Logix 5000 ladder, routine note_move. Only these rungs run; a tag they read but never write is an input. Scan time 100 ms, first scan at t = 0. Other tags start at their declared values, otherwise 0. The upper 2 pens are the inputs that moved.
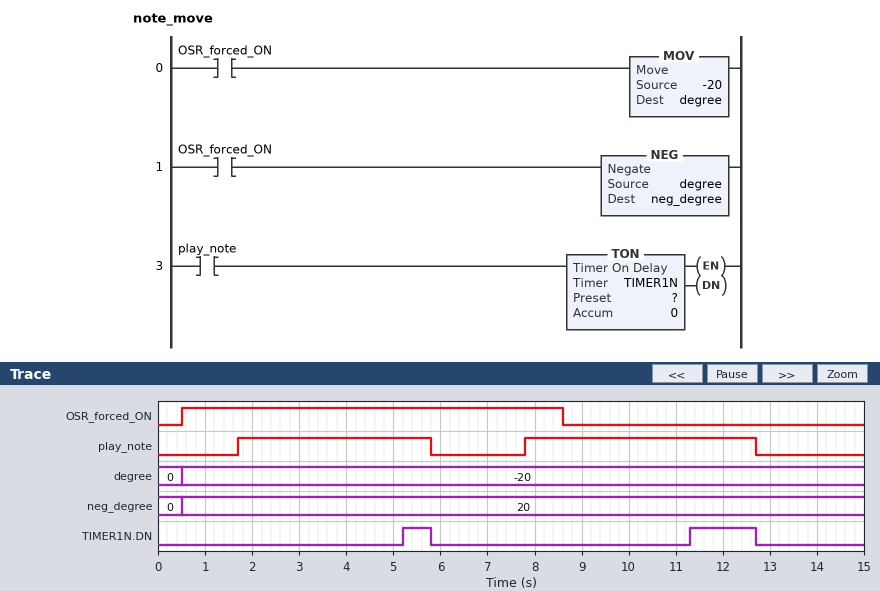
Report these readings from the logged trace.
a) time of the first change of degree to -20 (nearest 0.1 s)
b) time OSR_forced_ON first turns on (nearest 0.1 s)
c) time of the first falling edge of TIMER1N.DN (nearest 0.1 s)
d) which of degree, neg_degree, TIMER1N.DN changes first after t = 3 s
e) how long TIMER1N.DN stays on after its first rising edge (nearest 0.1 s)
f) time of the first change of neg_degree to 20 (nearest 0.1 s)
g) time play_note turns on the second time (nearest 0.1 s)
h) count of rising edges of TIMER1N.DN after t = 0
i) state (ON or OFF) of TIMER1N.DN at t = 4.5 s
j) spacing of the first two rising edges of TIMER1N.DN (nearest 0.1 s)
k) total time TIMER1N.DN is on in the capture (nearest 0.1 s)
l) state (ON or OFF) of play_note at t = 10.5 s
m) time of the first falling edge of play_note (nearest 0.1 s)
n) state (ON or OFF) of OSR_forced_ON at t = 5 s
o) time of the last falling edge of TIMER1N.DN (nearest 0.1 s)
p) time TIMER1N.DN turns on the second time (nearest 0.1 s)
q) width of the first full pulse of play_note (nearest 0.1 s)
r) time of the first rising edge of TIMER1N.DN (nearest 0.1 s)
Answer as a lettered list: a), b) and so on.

a) 0.5 s
b) 0.5 s
c) 5.8 s
d) TIMER1N.DN
e) 0.6 s
f) 0.5 s
g) 7.8 s
h) 2
i) OFF
j) 6.1 s
k) 2.0 s
l) ON
m) 5.8 s
n) ON
o) 12.7 s
p) 11.3 s
q) 4.1 s
r) 5.2 s
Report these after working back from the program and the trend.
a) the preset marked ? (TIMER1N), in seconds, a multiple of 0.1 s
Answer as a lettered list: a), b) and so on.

a) 3.5 s
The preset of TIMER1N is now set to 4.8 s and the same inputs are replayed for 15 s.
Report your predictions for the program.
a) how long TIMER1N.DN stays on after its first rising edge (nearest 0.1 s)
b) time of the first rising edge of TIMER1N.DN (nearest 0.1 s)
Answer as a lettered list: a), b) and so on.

a) 0.1 s
b) 12.6 s
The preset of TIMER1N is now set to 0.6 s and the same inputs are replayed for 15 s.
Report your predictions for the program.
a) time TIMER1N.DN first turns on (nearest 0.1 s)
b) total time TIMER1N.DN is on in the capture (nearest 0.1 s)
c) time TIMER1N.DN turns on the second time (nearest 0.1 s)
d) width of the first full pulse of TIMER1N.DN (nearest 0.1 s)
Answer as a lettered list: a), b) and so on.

a) 2.3 s
b) 7.8 s
c) 8.4 s
d) 3.5 s
